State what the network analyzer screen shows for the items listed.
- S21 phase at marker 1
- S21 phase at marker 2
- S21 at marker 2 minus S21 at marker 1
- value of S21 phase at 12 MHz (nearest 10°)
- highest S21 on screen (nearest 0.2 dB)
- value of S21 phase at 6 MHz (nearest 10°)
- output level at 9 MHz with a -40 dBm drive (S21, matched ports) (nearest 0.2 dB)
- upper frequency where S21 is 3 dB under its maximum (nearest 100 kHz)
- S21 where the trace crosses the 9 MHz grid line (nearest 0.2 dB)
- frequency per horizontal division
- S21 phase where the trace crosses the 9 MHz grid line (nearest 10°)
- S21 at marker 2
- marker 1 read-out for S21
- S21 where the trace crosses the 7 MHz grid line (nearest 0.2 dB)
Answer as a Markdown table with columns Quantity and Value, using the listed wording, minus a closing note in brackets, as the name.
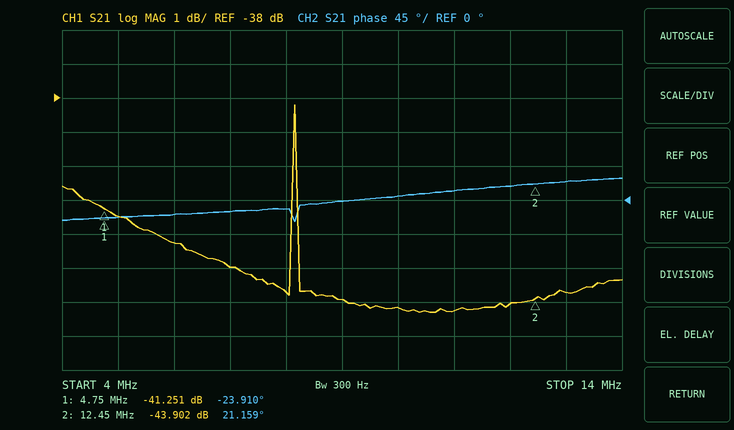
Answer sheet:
| Quantity | Value |
|---|---|
| S21 phase at marker 1 | -23.910° |
| S21 phase at marker 2 | 21.159° |
| S21 at marker 2 minus S21 at marker 1 | -2.651 dB |
| value of S21 phase at 12 MHz | 20° |
| highest S21 on screen | -38.2 dB |
| value of S21 phase at 6 MHz | -20° |
| output level at 9 MHz with a -40 dBm drive (S21, matched ports) | -84.0 dBm |
| upper frequency where S21 is 3 dB under its maximum | 8.2 MHz |
| S21 where the trace crosses the 9 MHz grid line | -44.0 dB |
| frequency per horizontal division | 1 MHz |
| S21 phase where the trace crosses the 9 MHz grid line | 0° |
| S21 at marker 2 | -43.902 dB |
| marker 1 read-out for S21 | -41.251 dB |
| S21 where the trace crosses the 7 MHz grid line | -43.0 dB |
